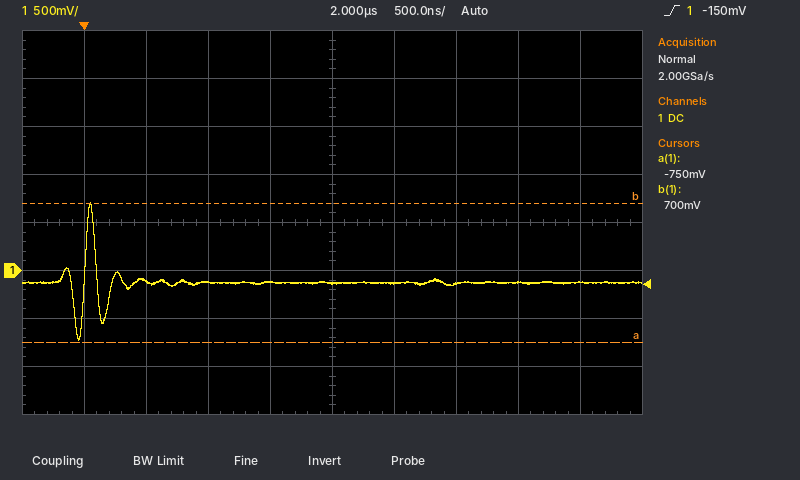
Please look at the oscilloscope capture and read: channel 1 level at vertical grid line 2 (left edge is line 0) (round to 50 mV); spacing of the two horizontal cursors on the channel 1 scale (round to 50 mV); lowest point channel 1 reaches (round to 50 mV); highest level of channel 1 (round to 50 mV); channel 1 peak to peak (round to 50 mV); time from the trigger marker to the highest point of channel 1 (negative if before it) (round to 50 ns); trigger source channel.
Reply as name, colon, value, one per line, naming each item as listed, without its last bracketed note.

channel 1 level at vertical grid line 2 (left edge is line 0): -100 mV
spacing of the two horizontal cursors on the channel 1 scale: 1.45 V
lowest point channel 1 reaches: -750 mV
highest level of channel 1: 700 mV
channel 1 peak to peak: 1.45 V
time from the trigger marker to the highest point of channel 1 (negative if before it): +50 ns
trigger source channel: channel 1
